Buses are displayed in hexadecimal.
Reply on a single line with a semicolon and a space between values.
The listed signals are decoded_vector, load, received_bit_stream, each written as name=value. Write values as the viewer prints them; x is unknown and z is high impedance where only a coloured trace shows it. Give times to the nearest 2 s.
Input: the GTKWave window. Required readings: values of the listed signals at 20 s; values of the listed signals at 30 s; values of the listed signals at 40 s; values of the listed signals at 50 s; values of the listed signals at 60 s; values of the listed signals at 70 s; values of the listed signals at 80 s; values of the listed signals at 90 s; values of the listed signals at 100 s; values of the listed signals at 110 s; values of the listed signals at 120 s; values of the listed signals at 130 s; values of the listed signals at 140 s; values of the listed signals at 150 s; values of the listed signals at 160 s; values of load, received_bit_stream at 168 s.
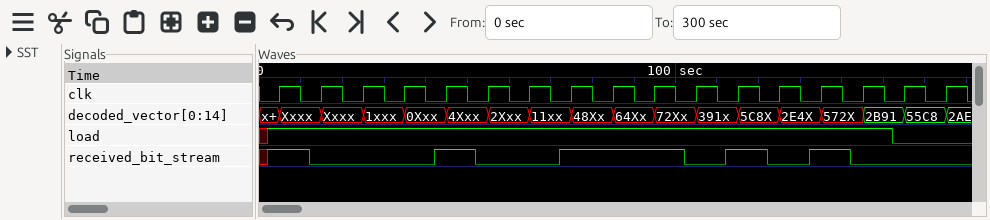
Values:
decoded_vector=Xxxx, load=1, received_bit_stream=0; decoded_vector=1xxx, load=1, received_bit_stream=0; decoded_vector=0Xxx, load=1, received_bit_stream=0; decoded_vector=4Xxx, load=1, received_bit_stream=1; decoded_vector=2Xxx, load=1, received_bit_stream=0; decoded_vector=11xx, load=1, received_bit_stream=0; decoded_vector=48Xx, load=1, received_bit_stream=1; decoded_vector=64Xx, load=1, received_bit_stream=1; decoded_vector=72Xx, load=1, received_bit_stream=1; decoded_vector=391x, load=1, received_bit_stream=0; decoded_vector=5C8X, load=1, received_bit_stream=1; decoded_vector=2E4X, load=1, received_bit_stream=0; decoded_vector=572X, load=1, received_bit_stream=1; decoded_vector=2B91, load=1, received_bit_stream=0; decoded_vector=55C8, load=0, received_bit_stream=0; load=0, received_bit_stream=0
